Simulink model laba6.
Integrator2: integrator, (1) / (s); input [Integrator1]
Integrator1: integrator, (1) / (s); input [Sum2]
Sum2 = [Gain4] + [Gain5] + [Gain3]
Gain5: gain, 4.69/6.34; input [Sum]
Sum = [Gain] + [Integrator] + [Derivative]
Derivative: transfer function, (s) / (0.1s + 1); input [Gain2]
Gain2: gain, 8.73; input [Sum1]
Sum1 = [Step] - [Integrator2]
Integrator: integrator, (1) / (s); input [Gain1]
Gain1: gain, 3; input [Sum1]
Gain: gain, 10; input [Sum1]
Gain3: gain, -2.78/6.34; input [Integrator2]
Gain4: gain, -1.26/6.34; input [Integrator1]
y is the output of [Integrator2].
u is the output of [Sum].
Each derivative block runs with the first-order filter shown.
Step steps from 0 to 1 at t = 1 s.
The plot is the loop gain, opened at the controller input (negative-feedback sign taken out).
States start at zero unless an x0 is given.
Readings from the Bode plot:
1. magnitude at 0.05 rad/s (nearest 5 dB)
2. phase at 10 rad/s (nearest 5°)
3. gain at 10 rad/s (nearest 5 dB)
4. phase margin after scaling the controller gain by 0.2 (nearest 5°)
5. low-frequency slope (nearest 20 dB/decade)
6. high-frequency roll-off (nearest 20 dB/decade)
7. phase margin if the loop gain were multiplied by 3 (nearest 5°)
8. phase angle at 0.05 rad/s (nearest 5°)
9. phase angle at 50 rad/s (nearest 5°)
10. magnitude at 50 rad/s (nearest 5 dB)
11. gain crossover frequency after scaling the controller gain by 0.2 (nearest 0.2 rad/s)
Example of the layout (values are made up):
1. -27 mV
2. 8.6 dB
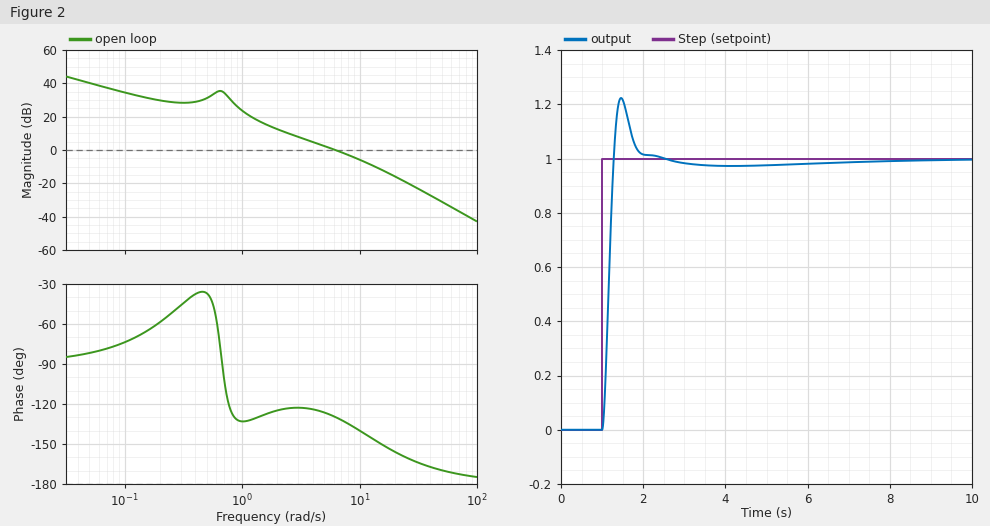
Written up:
1. 40 dB
2. -140°
3. -5 dB
4. 55°
5. -20 dB/decade
6. -40 dB/decade
7. 35°
8. -80°
9. -170°
10. -30 dB
11. 1.8 rad/s
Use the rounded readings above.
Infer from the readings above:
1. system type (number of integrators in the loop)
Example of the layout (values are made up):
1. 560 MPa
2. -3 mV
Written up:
1. 1
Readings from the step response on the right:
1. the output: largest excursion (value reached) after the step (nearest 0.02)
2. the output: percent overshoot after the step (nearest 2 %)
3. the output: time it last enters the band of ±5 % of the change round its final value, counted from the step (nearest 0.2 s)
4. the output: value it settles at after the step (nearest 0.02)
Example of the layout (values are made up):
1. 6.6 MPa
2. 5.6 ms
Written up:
1. 1.22
2. 22 %
3. 0.8 s
4. 1.00
